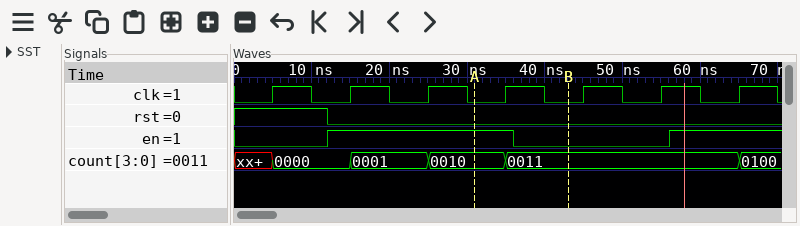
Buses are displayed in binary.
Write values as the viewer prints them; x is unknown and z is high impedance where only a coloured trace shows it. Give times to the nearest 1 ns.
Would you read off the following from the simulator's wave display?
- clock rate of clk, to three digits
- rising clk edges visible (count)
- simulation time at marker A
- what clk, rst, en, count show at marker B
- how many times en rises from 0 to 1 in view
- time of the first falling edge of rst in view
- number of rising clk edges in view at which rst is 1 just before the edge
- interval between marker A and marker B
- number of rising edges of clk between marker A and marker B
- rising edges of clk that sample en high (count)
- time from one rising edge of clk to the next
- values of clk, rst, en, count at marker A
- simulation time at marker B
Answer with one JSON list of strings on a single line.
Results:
["100 MHz", "7", "31 ns", "clk=0, rst=0, en=0, count=0011", "2", "12 ns", "1", "12 ns", "1", "4", "10 ns", "clk=0, rst=0, en=1, count=0010", "43 ns"]
